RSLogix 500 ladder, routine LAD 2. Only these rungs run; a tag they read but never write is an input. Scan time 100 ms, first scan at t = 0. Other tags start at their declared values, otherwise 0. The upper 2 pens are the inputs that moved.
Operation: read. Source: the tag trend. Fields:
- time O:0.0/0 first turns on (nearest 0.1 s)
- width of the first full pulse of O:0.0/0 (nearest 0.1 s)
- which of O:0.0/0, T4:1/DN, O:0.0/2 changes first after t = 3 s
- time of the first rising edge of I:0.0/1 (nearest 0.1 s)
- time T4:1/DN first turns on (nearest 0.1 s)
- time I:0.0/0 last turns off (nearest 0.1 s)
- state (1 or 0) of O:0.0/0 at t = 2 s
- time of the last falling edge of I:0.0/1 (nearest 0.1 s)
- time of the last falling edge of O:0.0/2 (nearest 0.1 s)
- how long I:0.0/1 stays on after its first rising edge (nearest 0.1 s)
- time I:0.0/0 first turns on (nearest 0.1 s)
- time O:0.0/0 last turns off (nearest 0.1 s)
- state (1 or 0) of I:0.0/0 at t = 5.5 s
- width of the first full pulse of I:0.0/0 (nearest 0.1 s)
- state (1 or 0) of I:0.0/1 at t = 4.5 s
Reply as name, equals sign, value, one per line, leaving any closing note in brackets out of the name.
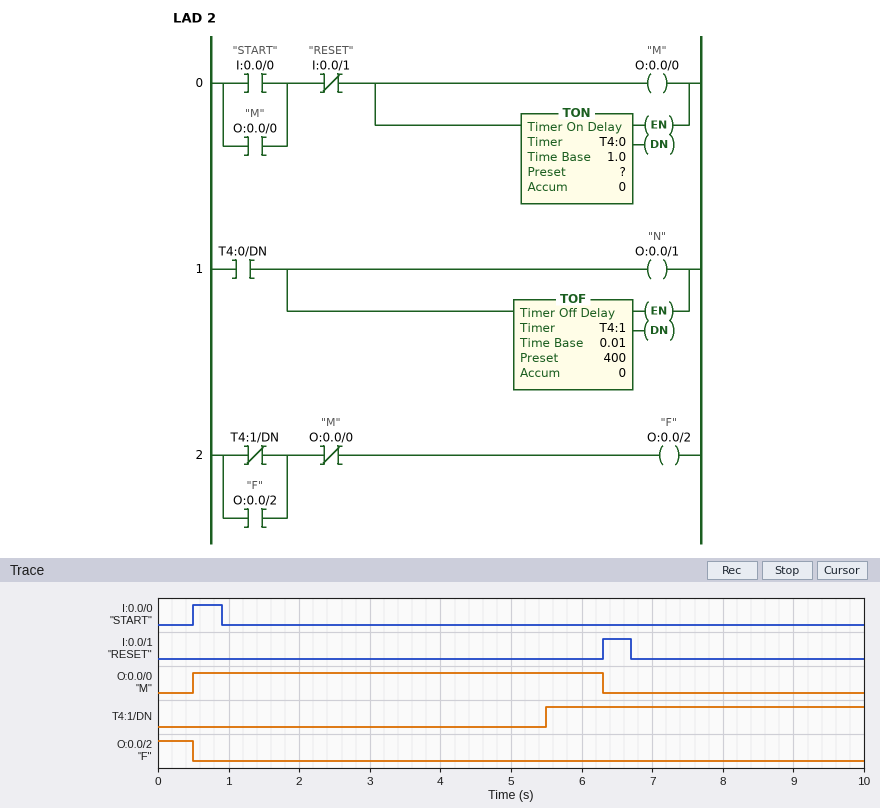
time O:0.0/0 first turns on = 0.5 s
width of the first full pulse of O:0.0/0 = 5.8 s
which of O:0.0/0, T4:1/DN, O:0.0/2 changes first after t = 3 s = T4:1/DN
time of the first rising edge of I:0.0/1 = 6.3 s
time T4:1/DN first turns on = 5.5 s
time I:0.0/0 last turns off = 0.9 s
state (1 or 0) of O:0.0/0 at t = 2 s = 1
time of the last falling edge of I:0.0/1 = 6.7 s
time of the last falling edge of O:0.0/2 = 0.5 s
how long I:0.0/1 stays on after its first rising edge = 0.4 s
time I:0.0/0 first turns on = 0.5 s
time O:0.0/0 last turns off = 6.3 s
state (1 or 0) of I:0.0/0 at t = 5.5 s = 0
width of the first full pulse of I:0.0/0 = 0.4 s
state (1 or 0) of I:0.0/1 at t = 4.5 s = 0
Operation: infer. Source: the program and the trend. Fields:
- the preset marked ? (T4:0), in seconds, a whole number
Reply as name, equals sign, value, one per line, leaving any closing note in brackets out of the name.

the preset marked ? (T4:0), in seconds, a whole number = 5 s
